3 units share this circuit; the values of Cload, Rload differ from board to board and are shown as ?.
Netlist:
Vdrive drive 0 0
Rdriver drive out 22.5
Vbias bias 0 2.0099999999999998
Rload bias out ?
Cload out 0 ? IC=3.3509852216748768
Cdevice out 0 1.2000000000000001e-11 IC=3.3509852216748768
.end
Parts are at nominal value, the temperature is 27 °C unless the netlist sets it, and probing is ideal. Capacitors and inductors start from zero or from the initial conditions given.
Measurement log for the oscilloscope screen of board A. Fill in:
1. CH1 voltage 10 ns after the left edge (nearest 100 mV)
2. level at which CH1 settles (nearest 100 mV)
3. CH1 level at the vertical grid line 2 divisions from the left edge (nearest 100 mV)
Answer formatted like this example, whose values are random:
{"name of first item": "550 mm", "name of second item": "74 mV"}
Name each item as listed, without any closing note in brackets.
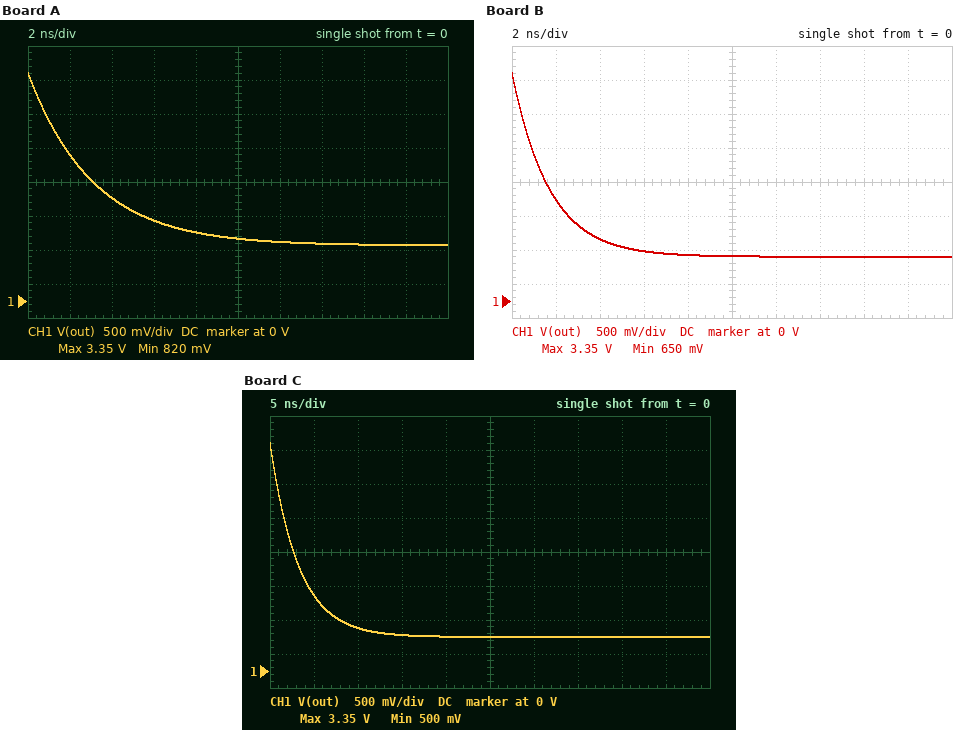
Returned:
{"CH1 voltage 10 ns after the left edge": "900 mV", "level at which CH1 settles": "800 mV", "CH1 level at the vertical grid line 2 divisions from the left edge": "1.5 V"}
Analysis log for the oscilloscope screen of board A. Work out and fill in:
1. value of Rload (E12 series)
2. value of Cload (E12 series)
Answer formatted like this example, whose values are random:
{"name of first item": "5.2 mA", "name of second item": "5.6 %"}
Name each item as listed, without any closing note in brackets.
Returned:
{"value of Rload": "33 Ω", "value of Cload": "220 pF"}
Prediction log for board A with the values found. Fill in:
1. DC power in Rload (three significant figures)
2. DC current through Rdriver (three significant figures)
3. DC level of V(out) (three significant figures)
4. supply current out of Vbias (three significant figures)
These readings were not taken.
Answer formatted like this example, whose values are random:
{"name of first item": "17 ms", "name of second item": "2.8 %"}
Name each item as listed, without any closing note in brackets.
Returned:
{"DC power in Rload": "43.3 mW", "DC current through Rdriver": "36.2 mA", "DC level of V(out)": "815 mV", "supply current out of Vbias": "36.2 mA"}
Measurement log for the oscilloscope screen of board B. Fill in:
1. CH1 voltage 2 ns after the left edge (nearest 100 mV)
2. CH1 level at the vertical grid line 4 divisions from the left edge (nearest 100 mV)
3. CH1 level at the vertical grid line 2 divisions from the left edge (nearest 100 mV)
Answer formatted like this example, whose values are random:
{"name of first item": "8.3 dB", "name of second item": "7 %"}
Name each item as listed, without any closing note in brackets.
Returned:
{"CH1 voltage 2 ns after the left edge": "1.5 V", "CH1 level at the vertical grid line 4 divisions from the left edge": "700 mV", "CH1 level at the vertical grid line 2 divisions from the left edge": "900 mV"}
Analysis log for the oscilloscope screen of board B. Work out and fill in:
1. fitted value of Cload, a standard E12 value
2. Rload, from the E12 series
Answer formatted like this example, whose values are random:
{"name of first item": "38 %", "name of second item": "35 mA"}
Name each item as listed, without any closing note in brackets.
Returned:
{"fitted value of Cload, a standard E12 value": "100 pF", "Rload, from the E12 series": "47 Ω"}
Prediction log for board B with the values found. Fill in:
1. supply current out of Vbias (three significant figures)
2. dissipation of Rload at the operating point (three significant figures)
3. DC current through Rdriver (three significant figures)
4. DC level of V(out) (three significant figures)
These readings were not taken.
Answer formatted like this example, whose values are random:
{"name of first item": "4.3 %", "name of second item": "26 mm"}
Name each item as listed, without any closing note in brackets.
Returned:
{"supply current out of Vbias": "28.9 mA", "dissipation of Rload at the operating point": "39.3 mW", "DC current through Rdriver": "28.9 mA", "DC level of V(out)": "651 mV"}
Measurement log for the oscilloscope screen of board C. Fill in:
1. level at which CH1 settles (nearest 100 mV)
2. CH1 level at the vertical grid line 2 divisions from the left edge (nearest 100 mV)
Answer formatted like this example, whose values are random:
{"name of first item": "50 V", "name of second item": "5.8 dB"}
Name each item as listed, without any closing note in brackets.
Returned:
{"level at which CH1 settles": "500 mV", "CH1 level at the vertical grid line 2 divisions from the left edge": "600 mV"}
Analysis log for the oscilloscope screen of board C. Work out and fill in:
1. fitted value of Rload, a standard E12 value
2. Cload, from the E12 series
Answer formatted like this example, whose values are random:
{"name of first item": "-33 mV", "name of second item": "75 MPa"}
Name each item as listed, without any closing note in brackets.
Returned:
{"fitted value of Rload, a standard E12 value": "68 Ω", "Cload, from the E12 series": "180 pF"}
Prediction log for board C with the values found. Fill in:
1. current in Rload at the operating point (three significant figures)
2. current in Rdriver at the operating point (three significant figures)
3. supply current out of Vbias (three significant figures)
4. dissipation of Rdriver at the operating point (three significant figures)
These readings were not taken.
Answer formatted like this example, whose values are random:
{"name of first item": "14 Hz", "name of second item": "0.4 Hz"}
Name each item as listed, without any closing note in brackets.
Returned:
{"current in Rload at the operating point": "22.2 mA", "current in Rdriver at the operating point": "22.2 mA", "supply current out of Vbias": "22.2 mA", "dissipation of Rdriver at the operating point": "11.1 mW"}
